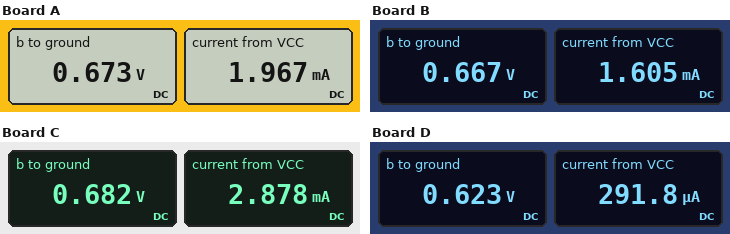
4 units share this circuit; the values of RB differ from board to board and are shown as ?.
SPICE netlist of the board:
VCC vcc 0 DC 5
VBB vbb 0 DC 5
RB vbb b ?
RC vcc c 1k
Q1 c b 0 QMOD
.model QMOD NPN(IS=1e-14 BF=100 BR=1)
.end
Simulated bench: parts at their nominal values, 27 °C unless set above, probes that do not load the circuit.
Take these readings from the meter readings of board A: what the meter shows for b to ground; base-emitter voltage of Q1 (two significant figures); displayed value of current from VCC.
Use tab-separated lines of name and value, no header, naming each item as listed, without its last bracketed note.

what the meter shows for b to ground	0.673 V
base-emitter voltage of Q1	670 mV
displayed value of current from VCC	1.967 mA
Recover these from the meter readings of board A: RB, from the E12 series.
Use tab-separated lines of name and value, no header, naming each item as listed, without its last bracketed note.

RB, from the E12 series	220 kΩ
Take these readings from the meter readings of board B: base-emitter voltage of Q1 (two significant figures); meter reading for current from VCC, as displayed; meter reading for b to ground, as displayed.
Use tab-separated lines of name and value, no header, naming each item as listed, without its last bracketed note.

base-emitter voltage of Q1	670 mV
meter reading for current from VCC, as displayed	1.605 mA
meter reading for b to ground, as displayed	0.667 V
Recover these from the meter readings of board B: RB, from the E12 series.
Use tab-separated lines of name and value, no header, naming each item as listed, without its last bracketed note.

RB, from the E12 series	270 kΩ
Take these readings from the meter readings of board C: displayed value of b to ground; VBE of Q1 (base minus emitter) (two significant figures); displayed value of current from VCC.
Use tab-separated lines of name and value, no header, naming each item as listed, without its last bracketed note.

displayed value of b to ground	0.682 V
VBE of Q1 (base minus emitter)	680 mV
displayed value of current from VCC	2.878 mA
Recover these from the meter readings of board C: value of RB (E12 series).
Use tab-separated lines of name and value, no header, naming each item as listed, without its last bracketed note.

value of RB	150 kΩ
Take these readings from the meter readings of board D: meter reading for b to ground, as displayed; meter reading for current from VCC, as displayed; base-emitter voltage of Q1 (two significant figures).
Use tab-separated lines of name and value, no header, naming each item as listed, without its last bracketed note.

meter reading for b to ground, as displayed	0.623 V
meter reading for current from VCC, as displayed	291.8 µA
base-emitter voltage of Q1	620 mV
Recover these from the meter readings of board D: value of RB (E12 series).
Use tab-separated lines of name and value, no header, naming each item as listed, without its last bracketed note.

value of RB	1.5 MΩ
